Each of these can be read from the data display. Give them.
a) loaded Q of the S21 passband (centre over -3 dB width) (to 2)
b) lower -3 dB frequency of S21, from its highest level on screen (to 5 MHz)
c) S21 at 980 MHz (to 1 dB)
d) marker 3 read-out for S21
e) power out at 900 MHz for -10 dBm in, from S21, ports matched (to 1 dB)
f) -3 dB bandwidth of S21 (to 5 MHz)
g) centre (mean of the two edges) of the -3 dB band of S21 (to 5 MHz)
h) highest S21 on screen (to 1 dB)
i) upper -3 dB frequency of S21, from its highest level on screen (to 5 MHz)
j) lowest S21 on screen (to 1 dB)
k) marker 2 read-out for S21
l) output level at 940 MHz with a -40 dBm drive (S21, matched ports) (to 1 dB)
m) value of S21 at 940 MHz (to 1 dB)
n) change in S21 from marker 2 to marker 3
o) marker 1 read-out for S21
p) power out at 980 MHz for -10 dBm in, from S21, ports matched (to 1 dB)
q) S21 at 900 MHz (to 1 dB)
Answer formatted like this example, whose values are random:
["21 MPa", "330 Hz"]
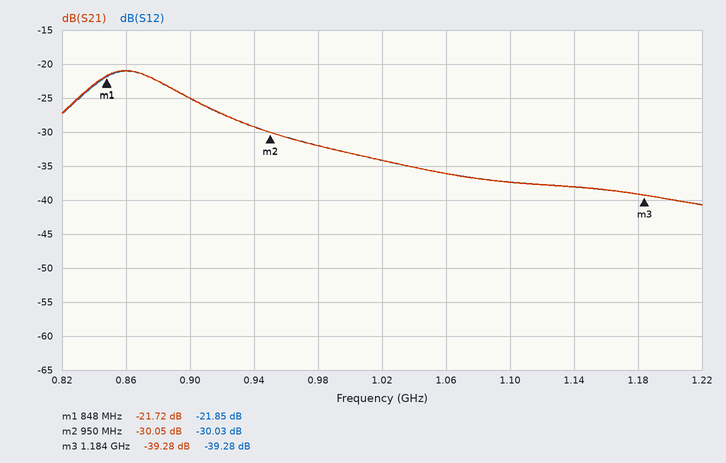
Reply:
["16", "835 MHz", "-32 dB", "-39.28 dB", "-35 dBm", "55 MHz", "865 MHz", "-21 dB", "890 MHz", "-41 dB", "-30.05 dB", "-69 dBm", "-29 dB", "-9.23 dB", "-21.72 dB", "-42 dBm", "-25 dB"]
